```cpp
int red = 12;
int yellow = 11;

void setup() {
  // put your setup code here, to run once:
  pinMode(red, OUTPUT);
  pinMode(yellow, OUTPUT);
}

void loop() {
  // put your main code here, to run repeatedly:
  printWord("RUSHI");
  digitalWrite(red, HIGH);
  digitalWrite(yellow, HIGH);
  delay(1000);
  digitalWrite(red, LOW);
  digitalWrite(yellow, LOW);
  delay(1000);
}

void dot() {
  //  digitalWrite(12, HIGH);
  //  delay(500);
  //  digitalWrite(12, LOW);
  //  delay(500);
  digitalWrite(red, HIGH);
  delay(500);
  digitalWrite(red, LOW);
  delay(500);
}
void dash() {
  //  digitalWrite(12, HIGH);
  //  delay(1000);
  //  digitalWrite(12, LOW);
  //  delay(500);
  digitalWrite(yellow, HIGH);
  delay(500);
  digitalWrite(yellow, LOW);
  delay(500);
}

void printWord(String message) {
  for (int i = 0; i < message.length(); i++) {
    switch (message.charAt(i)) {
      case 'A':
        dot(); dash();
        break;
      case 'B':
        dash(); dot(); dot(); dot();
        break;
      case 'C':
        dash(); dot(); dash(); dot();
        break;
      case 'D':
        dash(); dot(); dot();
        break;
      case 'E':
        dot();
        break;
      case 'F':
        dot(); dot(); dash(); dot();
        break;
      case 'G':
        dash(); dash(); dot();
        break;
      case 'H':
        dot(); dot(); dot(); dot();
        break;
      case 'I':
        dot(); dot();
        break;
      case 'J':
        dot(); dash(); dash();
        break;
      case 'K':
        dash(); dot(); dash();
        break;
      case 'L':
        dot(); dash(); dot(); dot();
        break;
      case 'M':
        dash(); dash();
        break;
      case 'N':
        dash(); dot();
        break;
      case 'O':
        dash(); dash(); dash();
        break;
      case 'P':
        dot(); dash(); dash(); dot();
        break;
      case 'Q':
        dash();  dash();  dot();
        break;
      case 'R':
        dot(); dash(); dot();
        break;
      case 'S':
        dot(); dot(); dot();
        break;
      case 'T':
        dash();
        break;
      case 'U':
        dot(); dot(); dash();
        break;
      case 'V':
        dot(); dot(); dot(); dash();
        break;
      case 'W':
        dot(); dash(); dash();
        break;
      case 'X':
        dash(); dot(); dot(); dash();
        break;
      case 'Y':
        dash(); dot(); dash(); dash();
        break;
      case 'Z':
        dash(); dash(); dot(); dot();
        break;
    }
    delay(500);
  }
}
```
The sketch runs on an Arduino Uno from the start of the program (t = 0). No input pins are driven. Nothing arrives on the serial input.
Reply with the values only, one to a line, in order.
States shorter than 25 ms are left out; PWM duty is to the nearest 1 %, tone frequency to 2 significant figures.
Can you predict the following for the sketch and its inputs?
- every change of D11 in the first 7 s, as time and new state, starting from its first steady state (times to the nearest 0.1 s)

0 s low; 1 s high; 1.5 s low; 5.5 s high; 6 s low
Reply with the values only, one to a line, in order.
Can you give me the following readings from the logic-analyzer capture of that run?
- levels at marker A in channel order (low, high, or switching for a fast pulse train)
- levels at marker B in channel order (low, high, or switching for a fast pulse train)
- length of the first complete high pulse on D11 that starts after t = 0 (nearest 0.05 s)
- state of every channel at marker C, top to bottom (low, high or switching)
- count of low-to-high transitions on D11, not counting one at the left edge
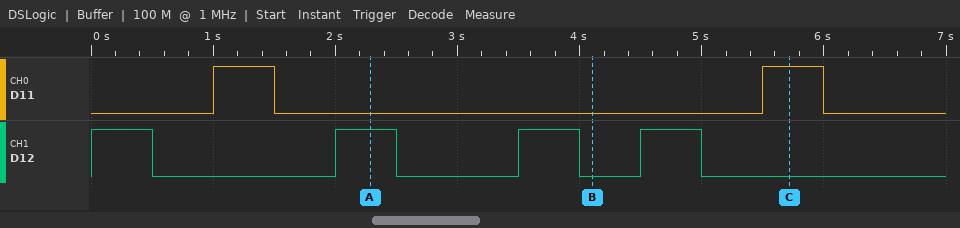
D11 low, D12 high
D11 low, D12 low
0.50 s
D11 high, D12 low
2
